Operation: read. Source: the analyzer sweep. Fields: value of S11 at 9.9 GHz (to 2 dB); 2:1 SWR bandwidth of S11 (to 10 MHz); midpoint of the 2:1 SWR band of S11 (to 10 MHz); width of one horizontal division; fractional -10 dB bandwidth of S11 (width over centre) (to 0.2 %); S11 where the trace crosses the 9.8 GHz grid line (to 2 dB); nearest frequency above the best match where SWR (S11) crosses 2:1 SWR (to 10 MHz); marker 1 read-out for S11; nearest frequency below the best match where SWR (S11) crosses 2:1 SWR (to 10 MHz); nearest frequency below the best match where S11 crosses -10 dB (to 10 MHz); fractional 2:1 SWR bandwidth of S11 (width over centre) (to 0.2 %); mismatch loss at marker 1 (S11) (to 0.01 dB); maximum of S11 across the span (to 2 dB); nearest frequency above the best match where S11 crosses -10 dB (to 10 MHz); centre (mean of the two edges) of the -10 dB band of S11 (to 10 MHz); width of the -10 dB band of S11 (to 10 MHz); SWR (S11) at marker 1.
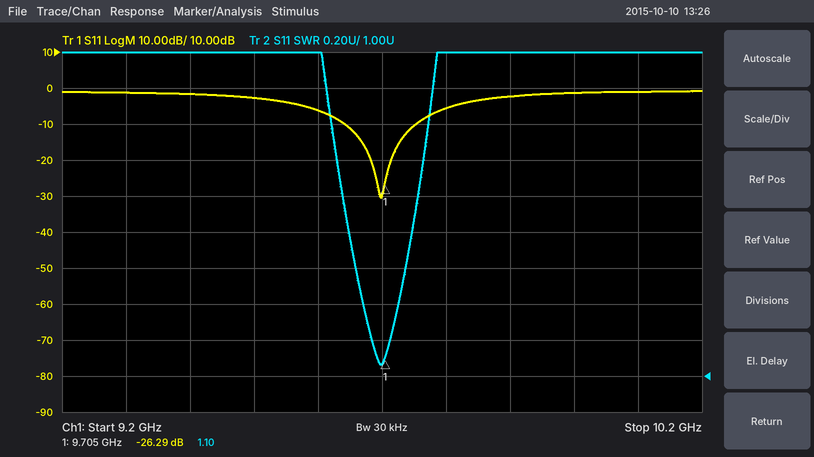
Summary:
-2 dB
120 MHz
9.70 GHz
100 MHz
1.2 %
-6 dB
9.76 GHz
-26.29 dB
9.64 GHz
9.64 GHz
1.2 %
0.01 dB
0 dB
9.75 GHz
9.70 GHz
110 MHz
1.10
